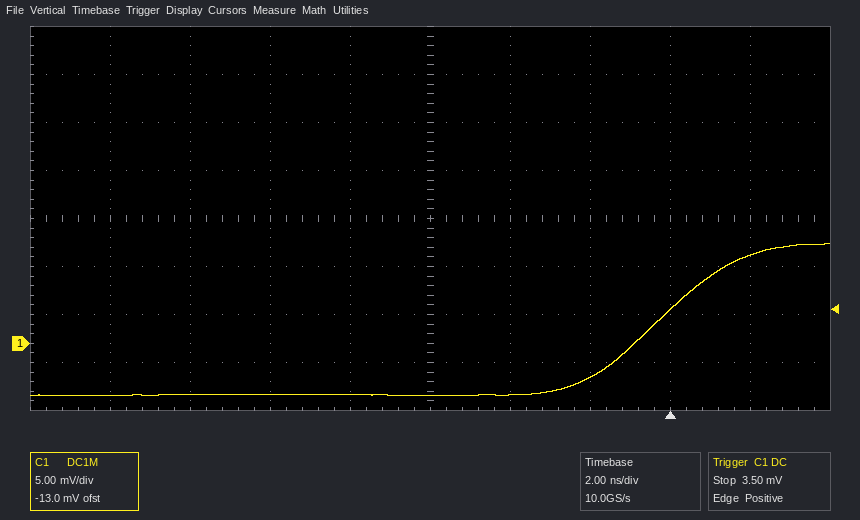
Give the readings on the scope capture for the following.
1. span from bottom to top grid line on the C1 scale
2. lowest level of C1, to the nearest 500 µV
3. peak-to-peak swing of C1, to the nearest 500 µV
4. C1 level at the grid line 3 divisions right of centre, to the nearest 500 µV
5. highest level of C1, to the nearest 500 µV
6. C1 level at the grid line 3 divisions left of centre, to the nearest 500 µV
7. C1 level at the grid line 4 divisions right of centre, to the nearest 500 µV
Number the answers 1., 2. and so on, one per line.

1. 40 mV
2. -5.5 mV
3. 16.0 mV
4. 3.5 mV
5. 10.5 mV
6. -5.5 mV
7. 9.0 mV
